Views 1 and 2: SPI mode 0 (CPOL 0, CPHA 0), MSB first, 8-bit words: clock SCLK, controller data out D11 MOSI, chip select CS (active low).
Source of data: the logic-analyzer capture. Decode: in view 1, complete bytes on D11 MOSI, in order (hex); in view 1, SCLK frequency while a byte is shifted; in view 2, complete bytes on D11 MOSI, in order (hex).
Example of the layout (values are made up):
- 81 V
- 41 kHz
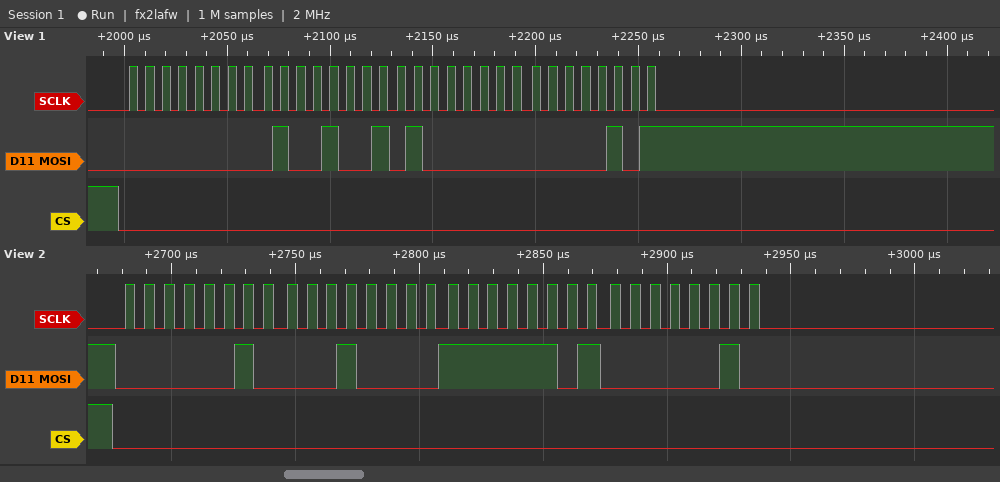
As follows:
- 00 49 40 05
- 125 kHz
- 02 10 FD 02
